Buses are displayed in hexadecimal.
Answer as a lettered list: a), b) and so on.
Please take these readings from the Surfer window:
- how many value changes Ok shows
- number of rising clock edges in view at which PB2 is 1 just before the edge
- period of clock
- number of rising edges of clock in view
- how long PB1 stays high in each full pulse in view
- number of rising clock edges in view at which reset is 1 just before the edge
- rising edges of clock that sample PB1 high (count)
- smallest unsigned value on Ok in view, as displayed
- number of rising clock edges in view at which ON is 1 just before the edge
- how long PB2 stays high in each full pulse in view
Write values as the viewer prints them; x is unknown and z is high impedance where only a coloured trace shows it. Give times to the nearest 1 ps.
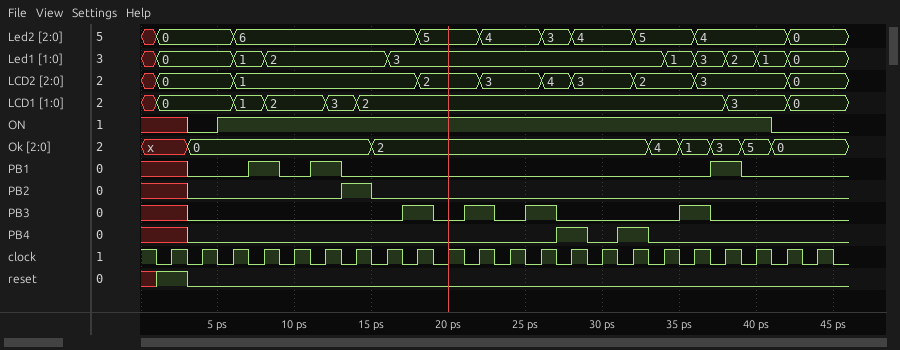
a) 7
b) 1
c) 2 ps
d) 22
e) 2 ps, 2 ps, 2 ps
f) 1
g) 3
h) 0
i) 18
j) 2 ps
